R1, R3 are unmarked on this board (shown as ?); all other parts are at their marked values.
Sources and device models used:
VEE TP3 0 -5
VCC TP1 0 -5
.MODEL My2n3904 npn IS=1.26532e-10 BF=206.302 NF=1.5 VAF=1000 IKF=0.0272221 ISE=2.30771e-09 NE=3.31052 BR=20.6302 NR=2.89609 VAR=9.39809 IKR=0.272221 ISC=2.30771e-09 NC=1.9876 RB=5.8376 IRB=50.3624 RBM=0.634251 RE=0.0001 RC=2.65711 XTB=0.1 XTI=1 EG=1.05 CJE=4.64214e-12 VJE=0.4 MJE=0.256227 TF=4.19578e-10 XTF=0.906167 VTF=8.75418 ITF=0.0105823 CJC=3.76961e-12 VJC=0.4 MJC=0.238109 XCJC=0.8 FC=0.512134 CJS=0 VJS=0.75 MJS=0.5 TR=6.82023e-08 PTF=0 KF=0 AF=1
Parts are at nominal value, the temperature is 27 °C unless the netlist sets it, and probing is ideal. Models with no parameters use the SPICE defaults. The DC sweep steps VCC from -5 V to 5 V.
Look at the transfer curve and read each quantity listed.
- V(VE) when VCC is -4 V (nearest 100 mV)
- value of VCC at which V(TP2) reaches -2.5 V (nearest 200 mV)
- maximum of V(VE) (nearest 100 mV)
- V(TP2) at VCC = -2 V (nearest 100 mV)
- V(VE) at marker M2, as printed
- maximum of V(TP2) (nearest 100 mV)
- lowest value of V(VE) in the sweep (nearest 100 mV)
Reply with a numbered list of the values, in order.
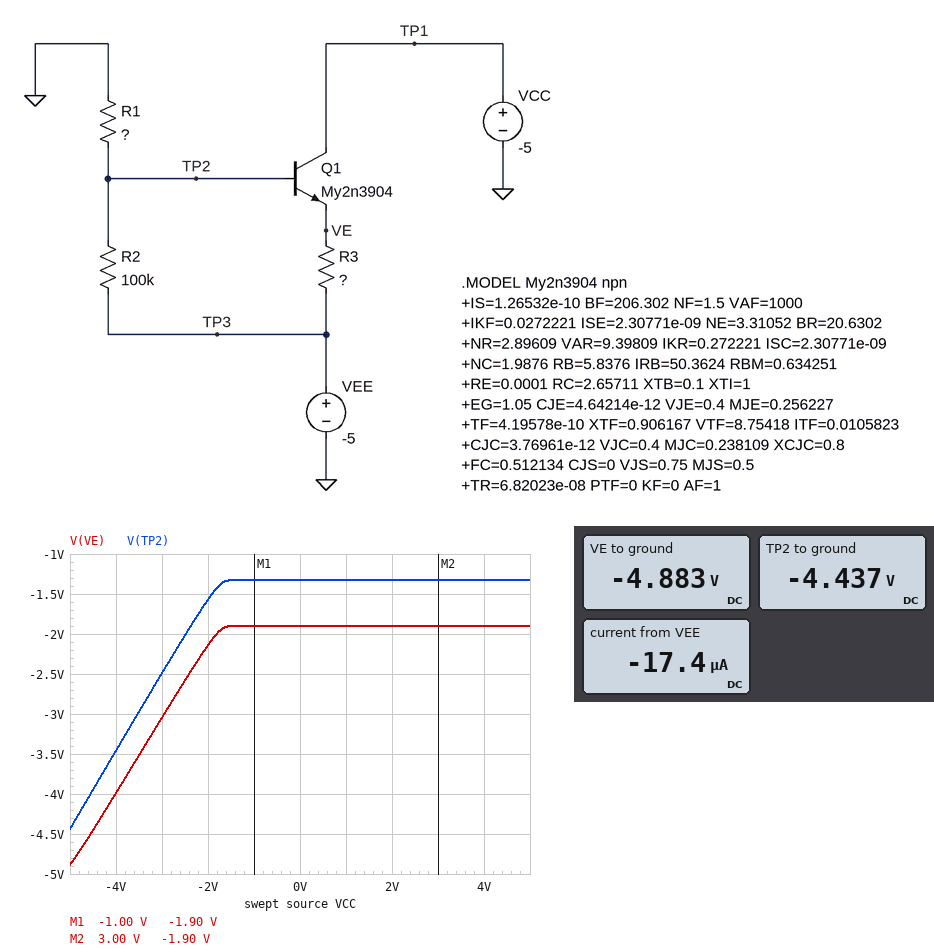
1. -4.0 V
2. -3.0 V
3. -1.9 V
4. -1.6 V
5. -1.90 V
6. -1.3 V
7. -4.9 V
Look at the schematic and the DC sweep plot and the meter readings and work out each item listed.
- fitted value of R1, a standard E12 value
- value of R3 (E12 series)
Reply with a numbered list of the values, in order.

1. 33 kΩ
2. 10 kΩ
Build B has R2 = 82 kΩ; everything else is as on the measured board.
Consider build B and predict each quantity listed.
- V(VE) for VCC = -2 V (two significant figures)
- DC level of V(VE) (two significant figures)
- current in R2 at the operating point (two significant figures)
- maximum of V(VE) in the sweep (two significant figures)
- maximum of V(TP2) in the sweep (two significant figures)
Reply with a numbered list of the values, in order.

1. -2.2 V
2. -4.9 V
3. 6.9 µA
4. -2.1 V
5. -1.5 V
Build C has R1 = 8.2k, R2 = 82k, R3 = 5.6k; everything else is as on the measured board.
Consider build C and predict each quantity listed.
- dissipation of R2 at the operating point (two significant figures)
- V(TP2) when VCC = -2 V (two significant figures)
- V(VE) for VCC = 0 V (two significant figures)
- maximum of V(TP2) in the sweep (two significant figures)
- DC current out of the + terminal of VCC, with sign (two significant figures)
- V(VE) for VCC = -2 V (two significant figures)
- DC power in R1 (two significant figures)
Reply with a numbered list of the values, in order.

1. 5.0 µW
2. -1.4 V
3. -1.1 V
4. -500 mV
5. -500 µA
6. -2.0 V
7. 2.3 mW
